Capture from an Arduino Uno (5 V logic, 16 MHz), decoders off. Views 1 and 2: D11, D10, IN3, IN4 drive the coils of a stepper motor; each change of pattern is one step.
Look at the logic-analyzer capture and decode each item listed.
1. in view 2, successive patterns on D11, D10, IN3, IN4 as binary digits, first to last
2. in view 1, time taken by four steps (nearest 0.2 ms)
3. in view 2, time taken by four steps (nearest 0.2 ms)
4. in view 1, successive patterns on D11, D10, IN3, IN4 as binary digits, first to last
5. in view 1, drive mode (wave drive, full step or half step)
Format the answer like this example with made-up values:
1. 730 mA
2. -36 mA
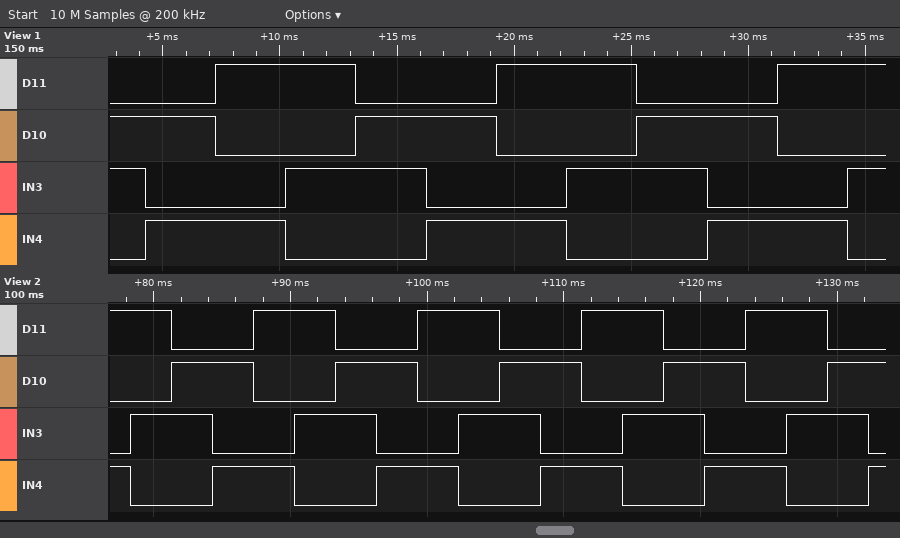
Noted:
1. 1001 1010 0110 0101 1001 1010 0110 0101 1001 1010 0110 0101 1001 1010 0110 0101 1001 1010 0110 0101
2. 12.0 ms
3. 12.0 ms
4. 0110 0101 1001 1010 0110 0101 1001 1010 0110 0101 1001 1010
5. full step
